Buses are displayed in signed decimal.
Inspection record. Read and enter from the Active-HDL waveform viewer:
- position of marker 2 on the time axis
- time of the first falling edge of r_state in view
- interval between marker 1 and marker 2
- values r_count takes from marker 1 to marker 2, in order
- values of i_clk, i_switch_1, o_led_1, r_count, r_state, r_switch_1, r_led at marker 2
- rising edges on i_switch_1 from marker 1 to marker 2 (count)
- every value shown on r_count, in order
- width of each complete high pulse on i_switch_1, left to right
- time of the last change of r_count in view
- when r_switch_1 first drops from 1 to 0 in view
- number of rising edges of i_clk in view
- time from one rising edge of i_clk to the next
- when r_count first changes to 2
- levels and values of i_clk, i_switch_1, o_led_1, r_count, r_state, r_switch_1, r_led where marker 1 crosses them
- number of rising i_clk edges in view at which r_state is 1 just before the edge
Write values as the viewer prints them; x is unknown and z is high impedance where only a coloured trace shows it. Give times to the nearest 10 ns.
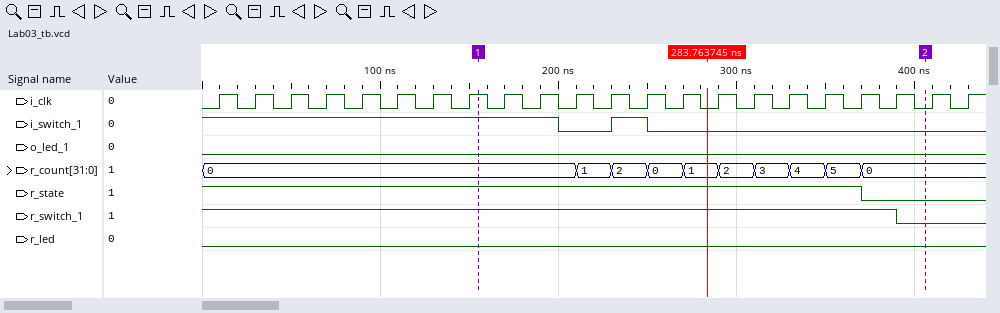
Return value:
410 ns
370 ns
250 ns
0, 1, 2, 0, 1, 2, 3, 4, 5, 0
i_clk=0, i_switch_1=0, o_led_1=0, r_count=0, r_state=0, r_switch_1=0, r_led=0
1
0, 1, 2, 0, 1, 2, 3, 4, 5, 0
20 ns
370 ns
390 ns
22
20 ns
230 ns
i_clk=1, i_switch_1=1, o_led_1=0, r_count=0, r_state=1, r_switch_1=1, r_led=0
19
